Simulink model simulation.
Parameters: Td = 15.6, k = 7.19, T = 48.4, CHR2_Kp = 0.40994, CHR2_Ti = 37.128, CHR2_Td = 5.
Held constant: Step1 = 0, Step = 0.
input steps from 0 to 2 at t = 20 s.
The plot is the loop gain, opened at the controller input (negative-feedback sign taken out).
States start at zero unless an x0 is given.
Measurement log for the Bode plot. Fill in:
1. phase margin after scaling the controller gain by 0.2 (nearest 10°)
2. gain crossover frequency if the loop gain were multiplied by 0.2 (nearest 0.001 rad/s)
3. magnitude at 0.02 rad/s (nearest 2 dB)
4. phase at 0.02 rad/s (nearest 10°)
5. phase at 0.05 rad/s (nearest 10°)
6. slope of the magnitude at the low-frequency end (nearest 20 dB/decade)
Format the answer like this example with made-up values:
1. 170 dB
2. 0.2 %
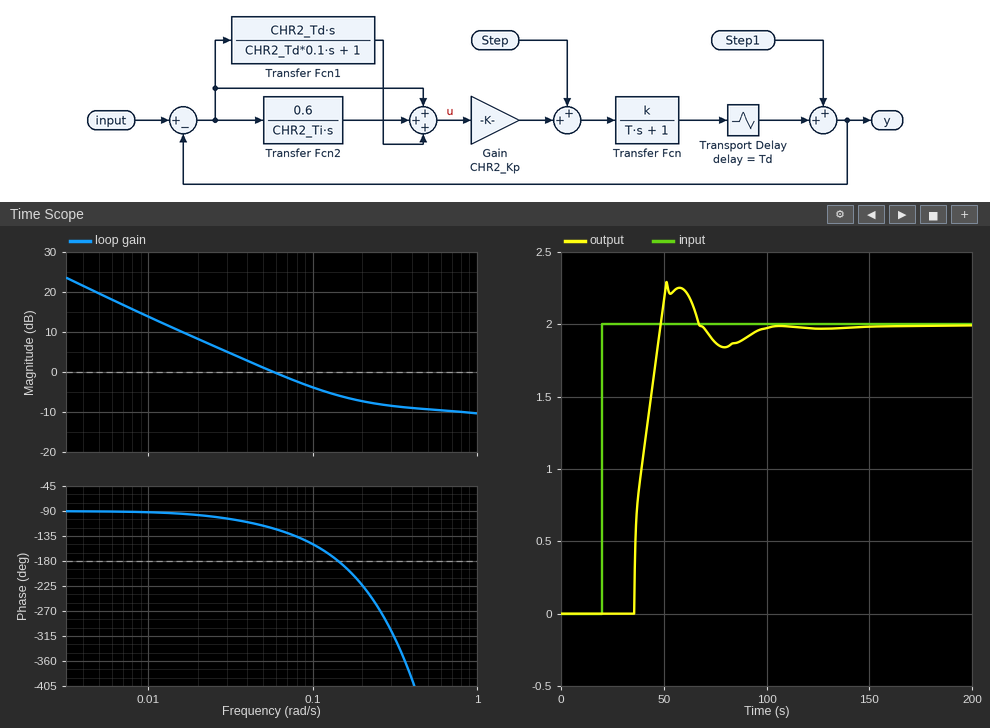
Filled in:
1. 90°
2. 0.010 rad/s
3. 8 dB
4. -100°
5. -120°
6. -20 dB/decade
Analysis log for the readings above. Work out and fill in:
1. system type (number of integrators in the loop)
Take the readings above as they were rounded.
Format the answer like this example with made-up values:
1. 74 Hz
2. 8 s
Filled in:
1. 1
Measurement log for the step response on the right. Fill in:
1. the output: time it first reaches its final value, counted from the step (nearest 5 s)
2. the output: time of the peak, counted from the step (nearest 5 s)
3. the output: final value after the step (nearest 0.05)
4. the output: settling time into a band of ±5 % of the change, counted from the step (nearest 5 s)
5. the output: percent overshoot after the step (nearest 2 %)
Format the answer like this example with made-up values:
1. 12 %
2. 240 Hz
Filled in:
1. 30 s
2. 30 s
3. 2.00
4. 70 s
5. 14 %
